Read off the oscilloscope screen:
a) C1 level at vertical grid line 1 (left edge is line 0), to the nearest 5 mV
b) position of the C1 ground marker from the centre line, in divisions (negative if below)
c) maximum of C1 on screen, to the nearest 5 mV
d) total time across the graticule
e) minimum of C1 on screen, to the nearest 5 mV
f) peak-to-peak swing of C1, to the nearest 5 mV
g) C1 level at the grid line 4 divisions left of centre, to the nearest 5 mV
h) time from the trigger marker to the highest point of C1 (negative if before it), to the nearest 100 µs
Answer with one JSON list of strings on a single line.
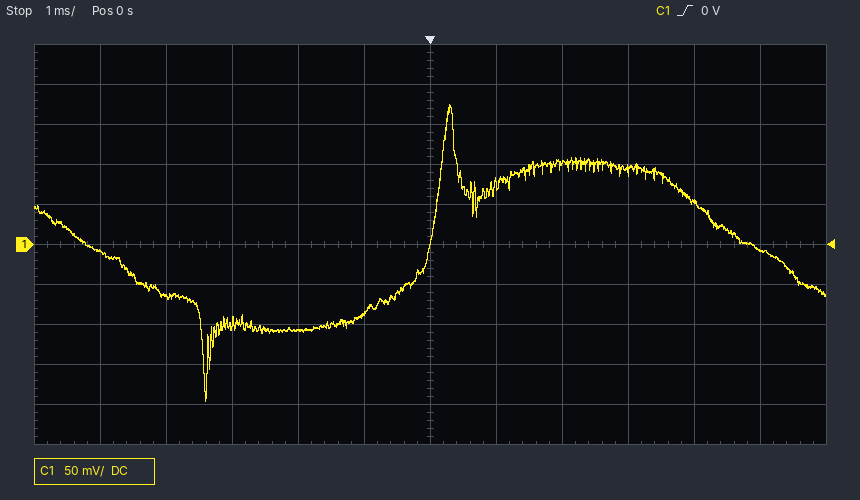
["-10 mV", "0.0 div", "175 mV", "12 ms", "-195 mV", "370 mV", "-65 mV", "+300 µs"]
